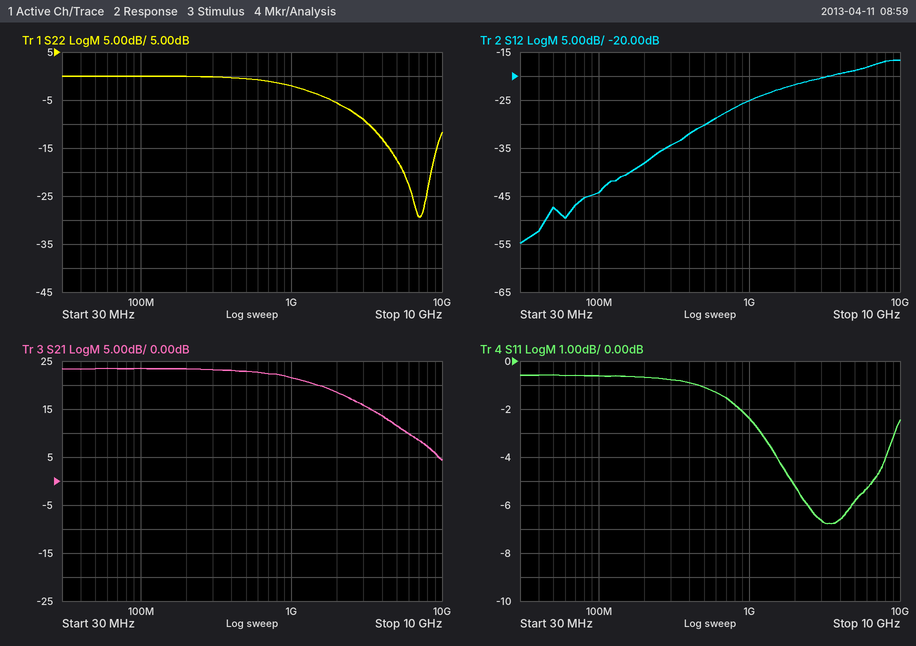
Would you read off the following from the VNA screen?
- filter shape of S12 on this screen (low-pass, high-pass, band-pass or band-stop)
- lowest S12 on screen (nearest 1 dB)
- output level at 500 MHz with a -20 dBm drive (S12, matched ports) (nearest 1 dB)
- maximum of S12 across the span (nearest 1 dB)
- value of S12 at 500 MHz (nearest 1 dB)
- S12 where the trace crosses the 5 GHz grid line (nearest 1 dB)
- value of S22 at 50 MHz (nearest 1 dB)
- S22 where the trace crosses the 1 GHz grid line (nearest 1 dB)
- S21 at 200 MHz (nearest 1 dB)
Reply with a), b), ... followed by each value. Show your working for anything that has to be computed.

a) high-pass
b) -55 dB
c) -20 dBm + (-30 dB) = -50 dBm
d) -17 dB
e) -30 dB
f) -19 dB
g) 0 dB
h) -2 dB
i) 23 dB
